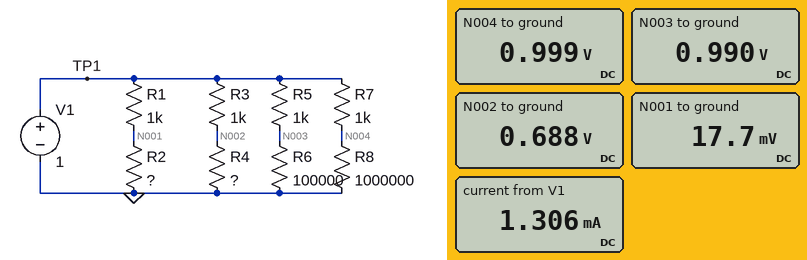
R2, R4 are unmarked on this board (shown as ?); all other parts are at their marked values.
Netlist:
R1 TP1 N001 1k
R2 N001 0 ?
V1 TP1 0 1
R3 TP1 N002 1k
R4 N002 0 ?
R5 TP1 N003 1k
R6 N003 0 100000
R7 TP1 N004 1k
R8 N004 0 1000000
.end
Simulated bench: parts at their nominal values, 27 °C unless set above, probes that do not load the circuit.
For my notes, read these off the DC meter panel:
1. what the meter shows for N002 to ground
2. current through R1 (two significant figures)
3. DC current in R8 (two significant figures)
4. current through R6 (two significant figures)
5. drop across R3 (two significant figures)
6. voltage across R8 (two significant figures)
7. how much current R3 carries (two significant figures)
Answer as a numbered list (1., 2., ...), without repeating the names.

1. 0.688 V
2. 980 µA
3. 1.0 µA
4. 9.9 µA
5. 310 mV
6. 1.0 V
7. 310 µA
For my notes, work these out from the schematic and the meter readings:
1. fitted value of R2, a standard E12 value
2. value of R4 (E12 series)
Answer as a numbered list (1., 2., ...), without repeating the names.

1. 18 Ω
2. 2.2 kΩ
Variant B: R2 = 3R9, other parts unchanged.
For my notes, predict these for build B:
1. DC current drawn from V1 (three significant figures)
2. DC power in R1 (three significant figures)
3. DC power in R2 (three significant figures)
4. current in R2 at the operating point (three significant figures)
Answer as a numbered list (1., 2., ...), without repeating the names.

1. 1.32 mA
2. 992 µW
3. 3.87 µW
4. 996 µA
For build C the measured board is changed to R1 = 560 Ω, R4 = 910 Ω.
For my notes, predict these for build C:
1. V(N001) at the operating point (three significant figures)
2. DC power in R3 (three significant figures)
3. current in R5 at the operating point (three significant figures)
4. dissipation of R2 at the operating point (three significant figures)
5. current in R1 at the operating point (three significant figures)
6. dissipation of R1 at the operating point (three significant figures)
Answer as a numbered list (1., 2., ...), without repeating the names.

1. 31.1 mV
2. 274 µW
3. 9.90 µA
4. 53.9 µW
5. 1.73 mA
6. 1.68 mW
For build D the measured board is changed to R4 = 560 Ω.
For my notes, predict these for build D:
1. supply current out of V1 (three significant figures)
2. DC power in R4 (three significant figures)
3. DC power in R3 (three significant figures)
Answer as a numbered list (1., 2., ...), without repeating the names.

1. 1.63 mA
2. 230 µW
3. 411 µW
